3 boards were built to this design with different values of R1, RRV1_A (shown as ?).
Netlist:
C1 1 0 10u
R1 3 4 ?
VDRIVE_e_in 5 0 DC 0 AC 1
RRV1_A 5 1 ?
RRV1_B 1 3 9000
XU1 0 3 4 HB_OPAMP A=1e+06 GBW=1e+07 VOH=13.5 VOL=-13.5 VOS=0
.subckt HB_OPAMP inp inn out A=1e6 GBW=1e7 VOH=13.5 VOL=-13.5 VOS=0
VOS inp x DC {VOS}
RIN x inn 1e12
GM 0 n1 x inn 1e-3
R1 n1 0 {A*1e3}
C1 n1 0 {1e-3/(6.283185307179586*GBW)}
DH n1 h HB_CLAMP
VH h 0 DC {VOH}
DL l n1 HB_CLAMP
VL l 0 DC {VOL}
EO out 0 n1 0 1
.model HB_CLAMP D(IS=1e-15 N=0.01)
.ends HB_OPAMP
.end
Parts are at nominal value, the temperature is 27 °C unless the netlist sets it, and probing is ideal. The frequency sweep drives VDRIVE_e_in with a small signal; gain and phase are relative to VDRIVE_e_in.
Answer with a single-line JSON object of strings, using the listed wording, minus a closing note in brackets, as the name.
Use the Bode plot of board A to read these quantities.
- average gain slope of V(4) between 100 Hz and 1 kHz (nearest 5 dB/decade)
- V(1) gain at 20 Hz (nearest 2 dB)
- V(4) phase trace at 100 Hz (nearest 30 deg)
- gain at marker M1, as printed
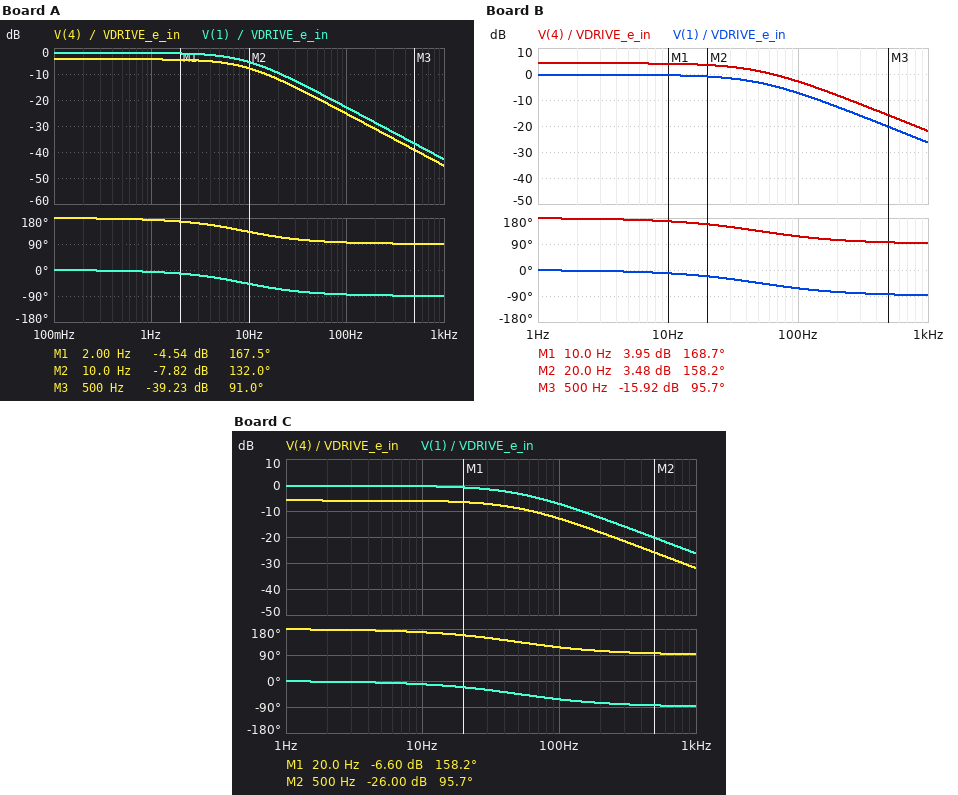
{"average gain slope of V(4) between 100 Hz and 1 kHz": "-20 dB/decade", "V(1) gain at 20 Hz": "-10 dB", "V(4) phase trace at 100 Hz": "90 deg", "gain at marker M1, as printed": "-4.54 dB"}
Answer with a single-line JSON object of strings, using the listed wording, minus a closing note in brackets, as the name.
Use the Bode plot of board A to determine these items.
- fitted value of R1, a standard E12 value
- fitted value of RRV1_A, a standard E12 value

{"fitted value of R1, a standard E12 value": "6.8 kΩ", "fitted value of RRV1_A, a standard E12 value": "2.2 kΩ"}
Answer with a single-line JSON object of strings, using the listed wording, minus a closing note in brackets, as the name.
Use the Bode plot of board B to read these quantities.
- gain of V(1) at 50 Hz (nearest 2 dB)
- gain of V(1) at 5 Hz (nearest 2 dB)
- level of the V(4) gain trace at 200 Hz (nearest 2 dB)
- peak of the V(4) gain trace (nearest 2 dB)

{"gain of V(1) at 50 Hz": "-4 dB", "gain of V(1) at 5 Hz": "0 dB", "level of the V(4) gain trace at 200 Hz": "-8 dB", "peak of the V(4) gain trace": "4 dB"}
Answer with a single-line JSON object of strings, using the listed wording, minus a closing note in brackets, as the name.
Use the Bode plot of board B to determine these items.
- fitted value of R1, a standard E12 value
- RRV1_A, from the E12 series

{"fitted value of R1, a standard E12 value": "15 kΩ", "RRV1_A, from the E12 series": "330 Ω"}
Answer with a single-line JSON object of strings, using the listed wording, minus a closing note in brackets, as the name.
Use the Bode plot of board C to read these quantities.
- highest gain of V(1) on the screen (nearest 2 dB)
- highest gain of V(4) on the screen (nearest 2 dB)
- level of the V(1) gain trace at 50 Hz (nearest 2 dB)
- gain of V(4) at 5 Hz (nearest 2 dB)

{"highest gain of V(1) on the screen": "0 dB", "highest gain of V(4) on the screen": "-6 dB", "level of the V(1) gain trace at 50 Hz": "-4 dB", "gain of V(4) at 5 Hz": "-6 dB"}
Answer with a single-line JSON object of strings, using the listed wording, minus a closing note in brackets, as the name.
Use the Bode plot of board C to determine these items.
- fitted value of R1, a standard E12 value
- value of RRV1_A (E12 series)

{"fitted value of R1, a standard E12 value": "4.7 kΩ", "value of RRV1_A": "330 Ω"}
